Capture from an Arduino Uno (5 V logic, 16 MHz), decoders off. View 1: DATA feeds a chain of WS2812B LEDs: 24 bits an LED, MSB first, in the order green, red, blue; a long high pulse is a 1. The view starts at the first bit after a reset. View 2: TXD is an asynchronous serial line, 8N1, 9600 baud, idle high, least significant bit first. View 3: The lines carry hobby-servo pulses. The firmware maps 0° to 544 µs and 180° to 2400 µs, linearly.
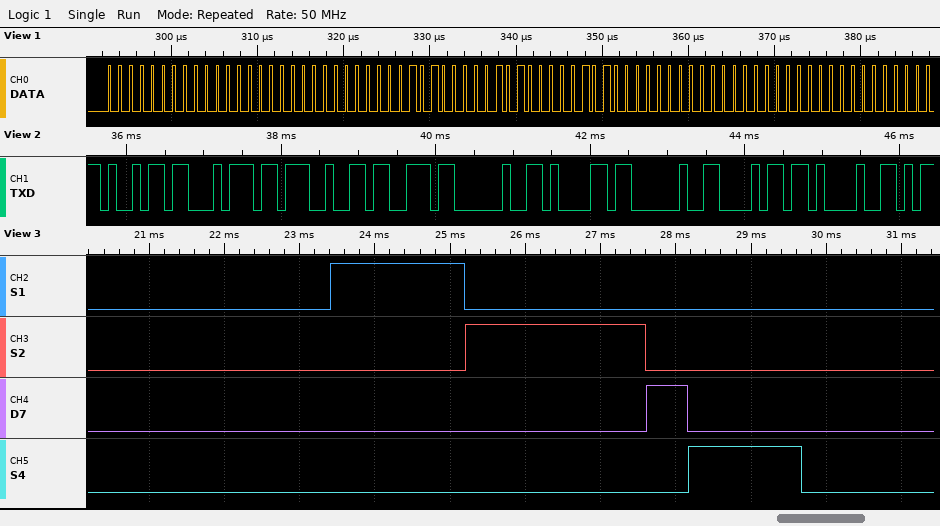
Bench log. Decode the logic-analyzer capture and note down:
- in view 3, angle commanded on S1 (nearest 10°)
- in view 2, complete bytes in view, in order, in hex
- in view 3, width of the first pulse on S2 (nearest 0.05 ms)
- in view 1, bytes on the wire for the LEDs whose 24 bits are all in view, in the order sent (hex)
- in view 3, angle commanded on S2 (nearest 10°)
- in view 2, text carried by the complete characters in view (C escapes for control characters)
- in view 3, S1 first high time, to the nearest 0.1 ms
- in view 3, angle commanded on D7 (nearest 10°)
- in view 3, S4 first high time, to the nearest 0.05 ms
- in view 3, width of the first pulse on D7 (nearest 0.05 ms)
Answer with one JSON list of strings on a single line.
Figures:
["120°", "69 74 27 73 20 61 20 68 21", "2.40 ms", "00 00 00 0A 0A 0A 00 00 00", "180°", "\"it's a h!\"", "1.8 ms", "0°", "1.50 ms", "0.55 ms"]
